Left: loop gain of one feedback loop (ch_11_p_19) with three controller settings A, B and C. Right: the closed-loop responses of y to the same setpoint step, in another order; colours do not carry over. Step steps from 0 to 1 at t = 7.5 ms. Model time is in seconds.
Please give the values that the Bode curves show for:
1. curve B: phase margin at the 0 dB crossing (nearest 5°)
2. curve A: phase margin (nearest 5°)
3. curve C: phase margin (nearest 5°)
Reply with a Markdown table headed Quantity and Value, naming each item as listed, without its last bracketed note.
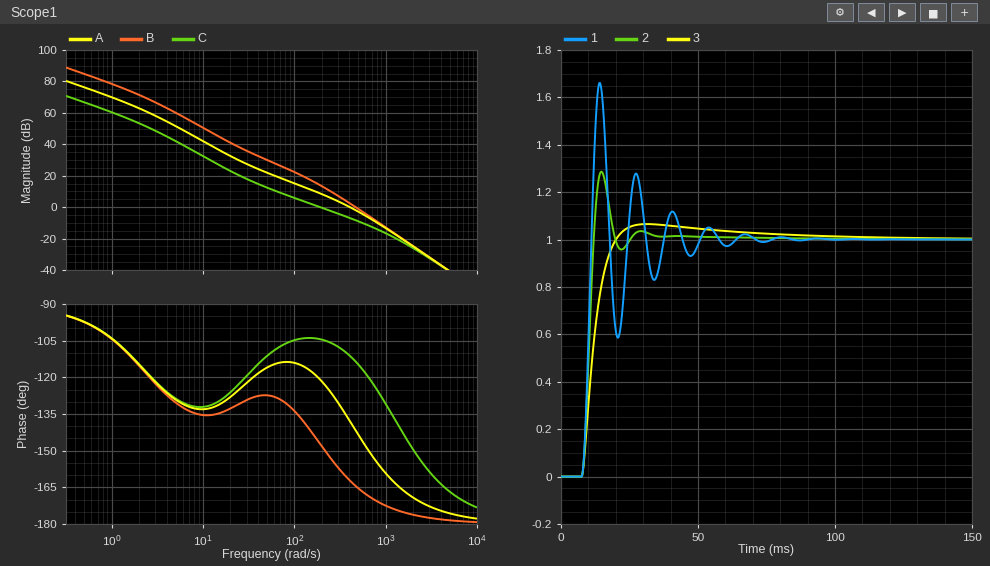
| Quantity | Value |
|---|---|
| curve B: phase margin at the 0 dB crossing | 15° |
| curve A: phase margin | 40° |
| curve C: phase margin | 75° |
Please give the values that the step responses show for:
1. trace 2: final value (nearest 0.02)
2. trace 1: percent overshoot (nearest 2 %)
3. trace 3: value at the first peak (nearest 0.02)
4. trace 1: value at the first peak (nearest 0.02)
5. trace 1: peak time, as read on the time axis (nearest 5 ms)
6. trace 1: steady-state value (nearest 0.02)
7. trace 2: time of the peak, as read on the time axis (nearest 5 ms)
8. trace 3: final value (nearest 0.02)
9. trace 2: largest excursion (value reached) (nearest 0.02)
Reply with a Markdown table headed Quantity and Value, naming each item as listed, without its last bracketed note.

| Quantity | Value |
|---|---|
| trace 2: final value | 1.00 |
| trace 1: percent overshoot | 66 % |
| trace 3: value at the first peak | 1.06 |
| trace 1: value at the first peak | 1.66 |
| trace 1: peak time, as read on the time axis | 15 ms |
| trace 1: steady-state value | 1.00 |
| trace 2: time of the peak, as read on the time axis | 15 ms |
| trace 3: final value | 1.00 |
| trace 2: largest excursion (value reached) | 1.28 |
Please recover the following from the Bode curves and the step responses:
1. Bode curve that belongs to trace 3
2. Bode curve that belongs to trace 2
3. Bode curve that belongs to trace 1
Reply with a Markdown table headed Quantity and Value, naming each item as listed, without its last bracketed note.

| Quantity | Value |
|---|---|
| Bode curve that belongs to trace 3 | C |
| Bode curve that belongs to trace 2 | A |
| Bode curve that belongs to trace 1 | B |
